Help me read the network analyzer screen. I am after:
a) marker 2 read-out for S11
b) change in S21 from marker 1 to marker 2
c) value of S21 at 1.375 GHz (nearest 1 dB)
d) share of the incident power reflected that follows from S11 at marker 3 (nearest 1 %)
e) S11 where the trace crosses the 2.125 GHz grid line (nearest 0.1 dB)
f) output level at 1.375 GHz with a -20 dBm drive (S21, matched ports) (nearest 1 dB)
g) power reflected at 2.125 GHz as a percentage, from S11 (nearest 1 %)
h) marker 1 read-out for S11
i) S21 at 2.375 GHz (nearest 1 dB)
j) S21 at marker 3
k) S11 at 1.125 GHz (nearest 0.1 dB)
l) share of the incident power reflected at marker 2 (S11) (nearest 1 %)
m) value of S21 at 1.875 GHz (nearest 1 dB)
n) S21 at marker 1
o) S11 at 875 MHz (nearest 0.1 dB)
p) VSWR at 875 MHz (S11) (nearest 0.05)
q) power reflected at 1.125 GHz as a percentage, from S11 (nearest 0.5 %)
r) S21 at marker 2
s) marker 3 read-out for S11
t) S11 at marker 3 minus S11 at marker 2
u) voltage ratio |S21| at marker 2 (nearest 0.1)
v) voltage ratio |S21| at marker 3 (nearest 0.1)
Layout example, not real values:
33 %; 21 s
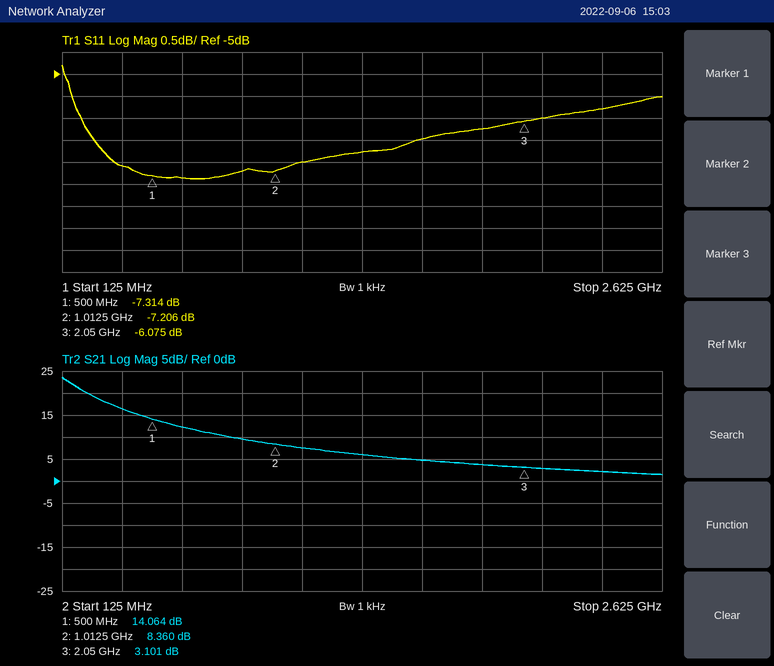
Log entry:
-7.206 dB; -5.704 dB; 6 dB; 25 %; -6.0 dB; -14 dBm; 25 %; -7.314 dB; 2 dB; 3.101 dB; -7.0 dB; 19 %; 4 dB; 14.064 dB; -7.2 dB; 2.55; 20.0 %; 8.360 dB; -6.075 dB; 1.131 dB; 2.6; 1.4
